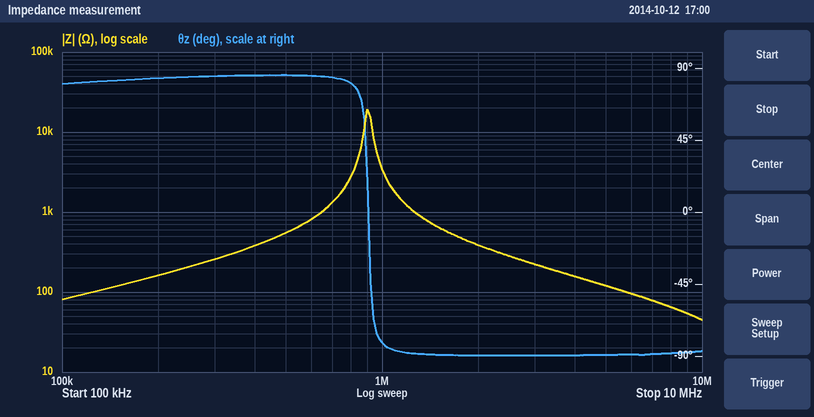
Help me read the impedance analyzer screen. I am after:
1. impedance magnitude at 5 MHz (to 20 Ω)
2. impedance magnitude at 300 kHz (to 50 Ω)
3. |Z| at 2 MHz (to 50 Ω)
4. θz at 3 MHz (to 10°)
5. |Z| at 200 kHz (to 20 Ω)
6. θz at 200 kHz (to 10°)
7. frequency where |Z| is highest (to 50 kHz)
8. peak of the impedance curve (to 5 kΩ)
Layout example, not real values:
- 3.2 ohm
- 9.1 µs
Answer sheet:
- 120 Ω
- 250 Ω
- 400 Ω
- -90°
- 160 Ω
- 80°
- 900 kHz
- 20 kΩ
